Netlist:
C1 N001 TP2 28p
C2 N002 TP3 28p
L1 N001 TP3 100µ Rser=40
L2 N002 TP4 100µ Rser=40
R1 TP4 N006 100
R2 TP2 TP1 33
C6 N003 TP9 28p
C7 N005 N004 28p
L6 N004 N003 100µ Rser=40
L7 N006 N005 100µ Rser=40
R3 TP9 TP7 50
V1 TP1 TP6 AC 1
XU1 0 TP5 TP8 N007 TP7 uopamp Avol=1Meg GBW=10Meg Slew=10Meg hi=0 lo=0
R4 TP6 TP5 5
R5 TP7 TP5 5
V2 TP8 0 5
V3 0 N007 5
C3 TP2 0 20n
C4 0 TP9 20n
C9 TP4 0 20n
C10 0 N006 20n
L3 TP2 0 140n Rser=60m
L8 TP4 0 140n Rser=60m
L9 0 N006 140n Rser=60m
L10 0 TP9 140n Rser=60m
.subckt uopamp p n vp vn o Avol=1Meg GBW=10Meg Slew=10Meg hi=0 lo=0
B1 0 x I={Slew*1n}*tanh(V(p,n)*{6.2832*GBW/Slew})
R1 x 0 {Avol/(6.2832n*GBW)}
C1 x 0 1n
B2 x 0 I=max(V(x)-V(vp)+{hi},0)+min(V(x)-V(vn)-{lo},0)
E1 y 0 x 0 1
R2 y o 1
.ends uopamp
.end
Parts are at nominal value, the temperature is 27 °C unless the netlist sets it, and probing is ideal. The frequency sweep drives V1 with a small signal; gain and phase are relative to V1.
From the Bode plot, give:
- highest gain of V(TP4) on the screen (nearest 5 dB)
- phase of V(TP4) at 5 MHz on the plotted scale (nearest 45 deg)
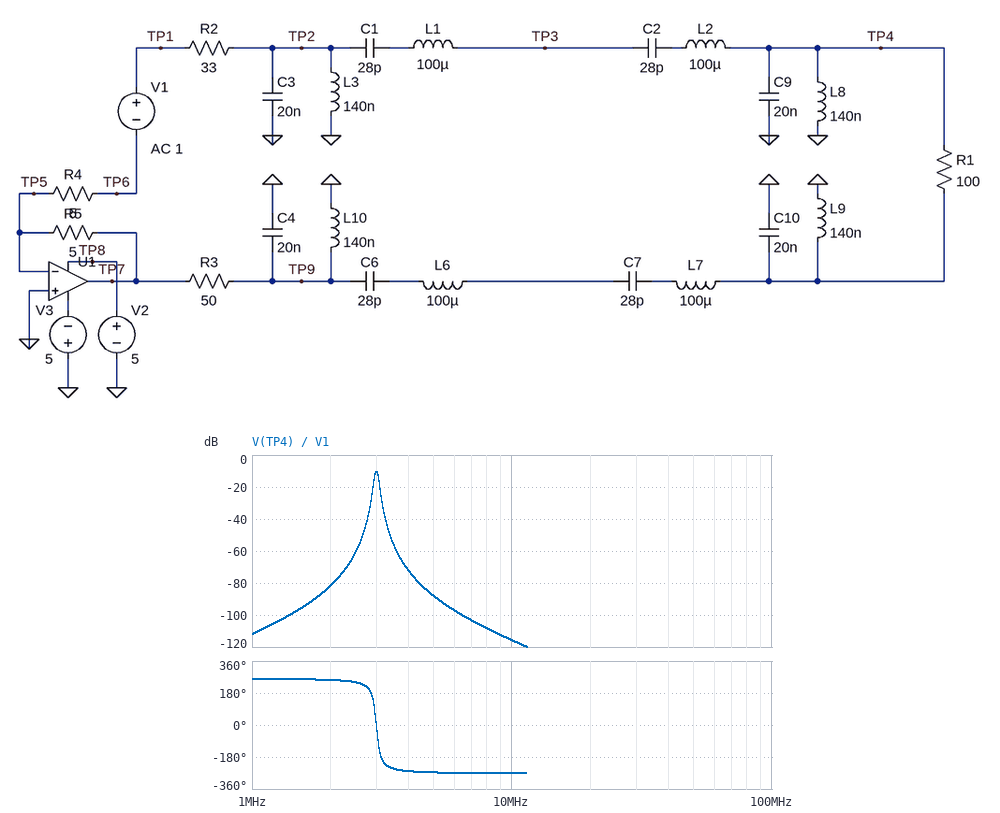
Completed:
-10 dB
-270 deg
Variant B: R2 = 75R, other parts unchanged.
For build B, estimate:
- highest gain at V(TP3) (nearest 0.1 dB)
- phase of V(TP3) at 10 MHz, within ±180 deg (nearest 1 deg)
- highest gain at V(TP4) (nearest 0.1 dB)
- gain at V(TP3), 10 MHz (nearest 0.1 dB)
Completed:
-9.7 dB
-91 deg
-13.7 dB
-45.6 dB
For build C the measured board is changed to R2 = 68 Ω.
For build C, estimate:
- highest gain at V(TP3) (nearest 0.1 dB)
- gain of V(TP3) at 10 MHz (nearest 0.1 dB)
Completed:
-9.3 dB
-44.8 dB
